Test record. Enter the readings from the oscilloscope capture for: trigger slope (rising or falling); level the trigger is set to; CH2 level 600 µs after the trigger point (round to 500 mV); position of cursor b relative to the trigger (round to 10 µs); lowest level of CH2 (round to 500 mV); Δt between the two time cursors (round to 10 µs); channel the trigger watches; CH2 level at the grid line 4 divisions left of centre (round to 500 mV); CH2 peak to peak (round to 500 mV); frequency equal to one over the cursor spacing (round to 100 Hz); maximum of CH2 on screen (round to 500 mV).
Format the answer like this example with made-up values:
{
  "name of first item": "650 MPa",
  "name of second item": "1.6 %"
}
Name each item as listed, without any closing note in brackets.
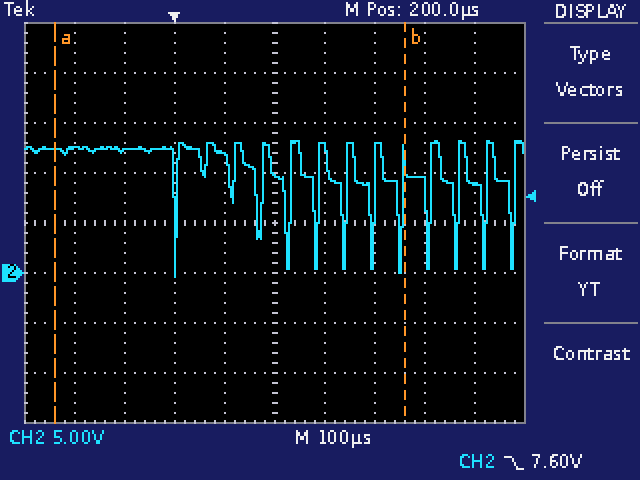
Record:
{
  "trigger slope": "falling",
  "level the trigger is set to": "7.60 V",
  "CH2 level 600 µs after the trigger point": "9.0 V",
  "position of cursor b relative to the trigger": "+460 µs",
  "lowest level of CH2": "-500 mV",
  "Δt between the two time cursors": "700 µs",
  "channel the trigger watches": "CH2",
  "CH2 level at the grid line 4 divisions left of centre": "12.5 V",
  "CH2 peak to peak": "13.5 V",
  "frequency equal to one over the cursor spacing": "1.4 kHz",
  "maximum of CH2 on screen": "13.0 V"
}
